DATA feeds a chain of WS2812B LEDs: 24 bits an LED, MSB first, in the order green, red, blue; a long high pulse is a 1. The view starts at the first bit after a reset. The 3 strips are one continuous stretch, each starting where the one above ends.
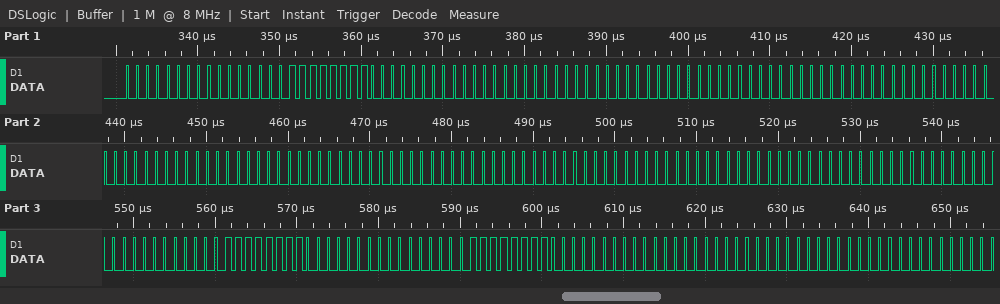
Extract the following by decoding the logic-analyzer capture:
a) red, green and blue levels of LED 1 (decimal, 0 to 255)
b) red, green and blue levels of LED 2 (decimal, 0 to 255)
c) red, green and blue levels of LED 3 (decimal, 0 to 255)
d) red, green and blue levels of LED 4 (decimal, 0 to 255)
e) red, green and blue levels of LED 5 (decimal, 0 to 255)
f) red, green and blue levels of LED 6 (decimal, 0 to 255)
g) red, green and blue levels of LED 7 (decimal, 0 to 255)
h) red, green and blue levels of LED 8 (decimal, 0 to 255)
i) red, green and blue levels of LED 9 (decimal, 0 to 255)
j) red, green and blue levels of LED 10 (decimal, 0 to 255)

0, 0, 255
0, 0, 0
0, 0, 0
0, 0, 0
0, 0, 0
0, 0, 0
0, 0, 0
0, 0, 255
0, 0, 255
0, 0, 0
